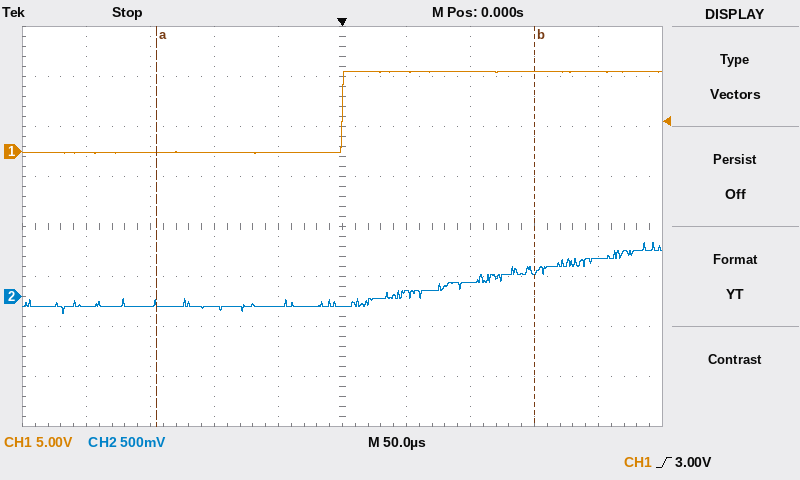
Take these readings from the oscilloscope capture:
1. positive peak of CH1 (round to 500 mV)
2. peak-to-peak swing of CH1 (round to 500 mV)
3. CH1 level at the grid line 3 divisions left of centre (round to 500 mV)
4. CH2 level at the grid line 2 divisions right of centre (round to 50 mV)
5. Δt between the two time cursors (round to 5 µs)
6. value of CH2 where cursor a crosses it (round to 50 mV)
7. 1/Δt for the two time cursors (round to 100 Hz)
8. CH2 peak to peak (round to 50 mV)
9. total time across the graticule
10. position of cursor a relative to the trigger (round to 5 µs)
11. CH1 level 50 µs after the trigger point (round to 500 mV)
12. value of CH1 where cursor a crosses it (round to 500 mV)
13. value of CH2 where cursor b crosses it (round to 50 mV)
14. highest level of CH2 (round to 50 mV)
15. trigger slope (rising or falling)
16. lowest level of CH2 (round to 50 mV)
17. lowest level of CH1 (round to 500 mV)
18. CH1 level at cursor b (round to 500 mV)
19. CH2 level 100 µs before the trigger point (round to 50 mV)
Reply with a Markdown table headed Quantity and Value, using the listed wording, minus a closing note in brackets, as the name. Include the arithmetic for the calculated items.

| Quantity | Value |
|---|---|
| positive peak of CH1 | 8.0 V |
| peak-to-peak swing of CH1 | 8.0 V − (0.0 V) = 8.0 V |
| CH1 level at the grid line 3 divisions left of centre | 0.0 V |
| CH2 level at the grid line 2 divisions right of centre | 150 mV |
| Δt between the two time cursors | 295 µs |
| value of CH2 where cursor a crosses it | -50 mV |
| 1/Δt for the two time cursors | 1 / 295 µs ≈ 3.4 kHz |
| CH2 peak to peak | 550 mV − (-150 mV) = 700 mV |
| total time across the graticule | 500 µs |
| position of cursor a relative to the trigger | -145 µs |
| CH1 level 50 µs after the trigger point | 8.0 V |
| value of CH1 where cursor a crosses it | 0.0 V |
| value of CH2 where cursor b crosses it | 250 mV |
| highest level of CH2 | 550 mV |
| trigger slope | rising |
| lowest level of CH2 | -150 mV |
| lowest level of CH1 | 0.0 V |
| CH1 level at cursor b | 8.0 V |
| CH2 level 100 µs before the trigger point | -100 mV |
